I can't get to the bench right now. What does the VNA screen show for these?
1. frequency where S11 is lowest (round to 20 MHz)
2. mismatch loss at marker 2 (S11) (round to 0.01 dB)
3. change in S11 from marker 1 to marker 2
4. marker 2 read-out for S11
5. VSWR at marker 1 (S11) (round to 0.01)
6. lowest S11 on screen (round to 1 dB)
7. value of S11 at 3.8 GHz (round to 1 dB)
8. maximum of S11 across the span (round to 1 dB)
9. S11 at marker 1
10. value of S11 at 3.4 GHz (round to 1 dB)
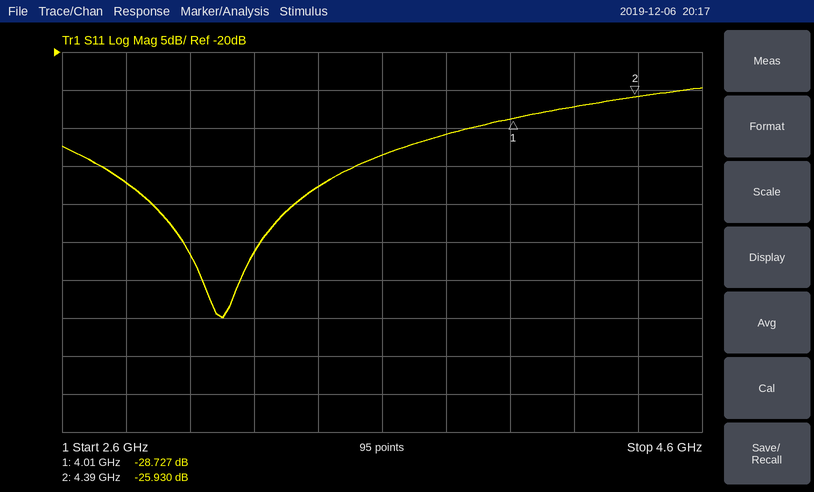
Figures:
3.10 GHz
0.01 dB
2.797 dB
-25.930 dB
1.08
-55 dB
-31 dB
-25 dB
-28.727 dB
-38 dB
